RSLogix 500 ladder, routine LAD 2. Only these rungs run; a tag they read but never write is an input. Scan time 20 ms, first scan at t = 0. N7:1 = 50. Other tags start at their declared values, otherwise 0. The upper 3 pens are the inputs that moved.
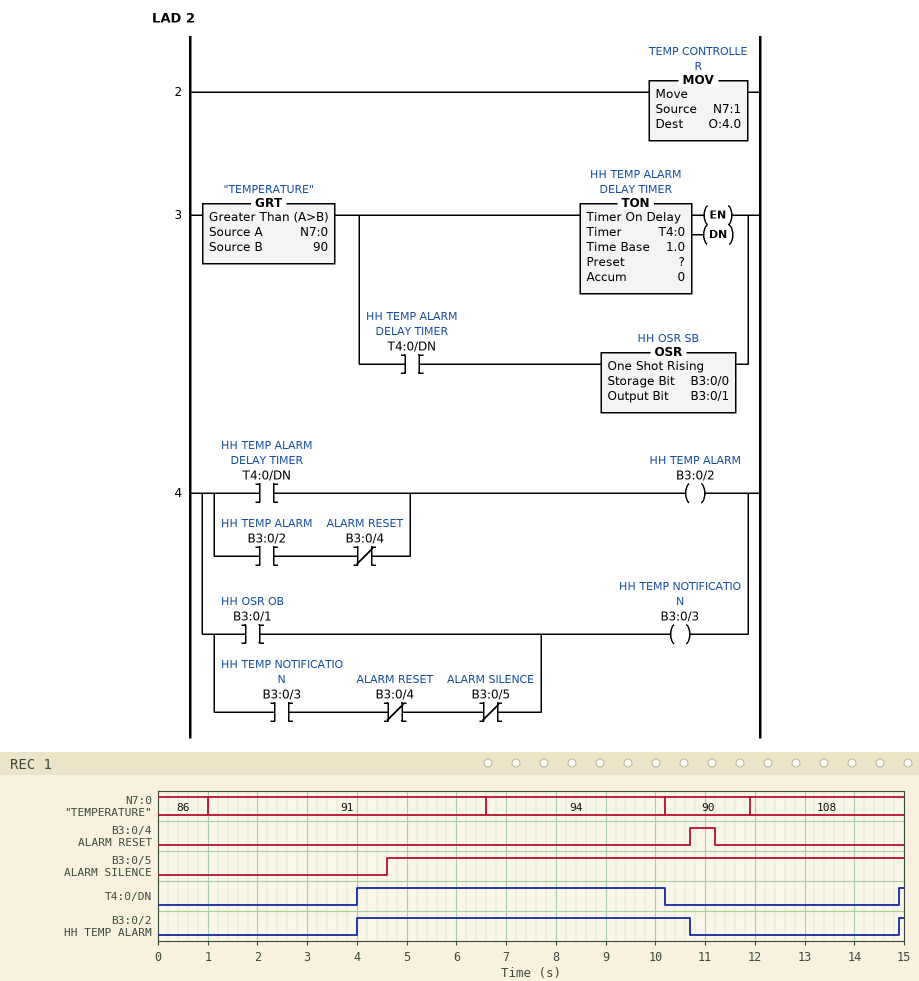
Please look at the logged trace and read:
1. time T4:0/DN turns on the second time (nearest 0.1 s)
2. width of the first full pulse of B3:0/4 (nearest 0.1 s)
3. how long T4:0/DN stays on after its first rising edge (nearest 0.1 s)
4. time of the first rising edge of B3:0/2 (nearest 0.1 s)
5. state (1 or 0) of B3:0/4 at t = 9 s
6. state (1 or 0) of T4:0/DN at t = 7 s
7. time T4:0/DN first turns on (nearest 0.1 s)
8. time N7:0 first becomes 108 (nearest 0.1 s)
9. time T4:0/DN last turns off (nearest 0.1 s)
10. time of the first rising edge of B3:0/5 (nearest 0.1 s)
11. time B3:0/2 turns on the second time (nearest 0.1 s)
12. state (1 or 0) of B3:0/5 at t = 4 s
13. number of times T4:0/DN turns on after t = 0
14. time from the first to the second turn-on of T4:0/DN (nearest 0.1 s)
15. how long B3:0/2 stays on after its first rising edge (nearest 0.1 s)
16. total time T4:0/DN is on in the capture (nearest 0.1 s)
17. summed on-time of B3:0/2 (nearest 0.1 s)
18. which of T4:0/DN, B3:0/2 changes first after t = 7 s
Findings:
14.9 s
0.5 s
6.2 s
4.0 s
0
1
4.0 s
11.9 s
10.2 s
4.6 s
14.9 s
0
2
10.9 s
6.7 s
6.3 s
6.8 s
T4:0/DN
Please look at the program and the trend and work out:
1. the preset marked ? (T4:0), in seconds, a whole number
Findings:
3 s
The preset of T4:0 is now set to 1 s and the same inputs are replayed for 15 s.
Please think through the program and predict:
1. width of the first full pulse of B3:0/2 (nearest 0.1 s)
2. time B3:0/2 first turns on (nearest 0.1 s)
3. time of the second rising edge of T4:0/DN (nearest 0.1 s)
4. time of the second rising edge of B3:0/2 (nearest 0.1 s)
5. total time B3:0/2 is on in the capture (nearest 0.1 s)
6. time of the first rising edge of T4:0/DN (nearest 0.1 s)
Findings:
8.7 s
2.0 s
12.9 s
12.9 s
10.8 s
2.0 s
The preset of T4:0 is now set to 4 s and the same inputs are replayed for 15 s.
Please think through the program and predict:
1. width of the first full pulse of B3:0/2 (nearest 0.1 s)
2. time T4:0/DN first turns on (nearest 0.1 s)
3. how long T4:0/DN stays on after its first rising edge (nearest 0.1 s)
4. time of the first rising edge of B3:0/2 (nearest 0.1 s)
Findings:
5.7 s
5.0 s
5.2 s
5.0 s
